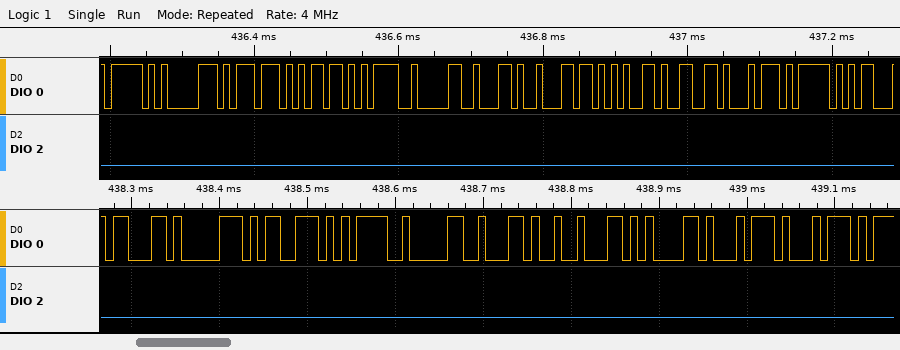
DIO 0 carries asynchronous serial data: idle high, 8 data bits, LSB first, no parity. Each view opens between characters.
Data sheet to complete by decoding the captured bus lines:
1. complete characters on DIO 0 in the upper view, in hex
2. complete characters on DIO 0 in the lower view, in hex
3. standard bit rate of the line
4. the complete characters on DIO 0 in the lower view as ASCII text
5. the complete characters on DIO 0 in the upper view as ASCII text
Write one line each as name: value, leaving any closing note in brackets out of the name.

complete characters on DIO 0 in the upper view, in hex: 5F, 70, 77, 6D, 3D, 30, 2C, 6C, 65, 66, 74, 5F
complete characters on DIO 0 in the lower view, in hex: 63, 70, 73, 3D, 30, 2C, 62, 61, 74, 74
standard bit rate of the line: 115200 baud
the complete characters on DIO 0 in the lower view as ASCII text: "cps=0,batt"
the complete characters on DIO 0 in the upper view as ASCII text: "_pwm=0,left_"
